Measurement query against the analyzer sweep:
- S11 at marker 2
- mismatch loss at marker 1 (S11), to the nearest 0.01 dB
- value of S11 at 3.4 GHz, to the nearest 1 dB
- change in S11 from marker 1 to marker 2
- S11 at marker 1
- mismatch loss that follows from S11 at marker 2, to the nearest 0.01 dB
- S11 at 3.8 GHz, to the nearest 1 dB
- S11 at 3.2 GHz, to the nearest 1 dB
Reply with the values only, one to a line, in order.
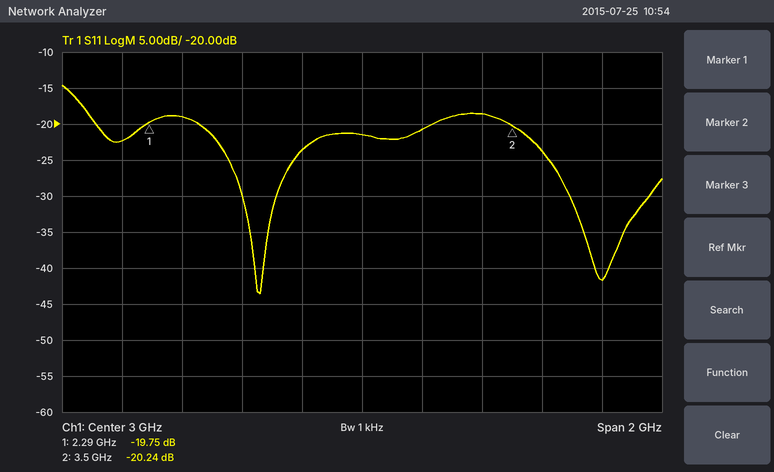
-20.24 dB
0.05 dB
-19 dB
-0.49 dB
-19.75 dB
0.04 dB
-42 dB
-21 dB
